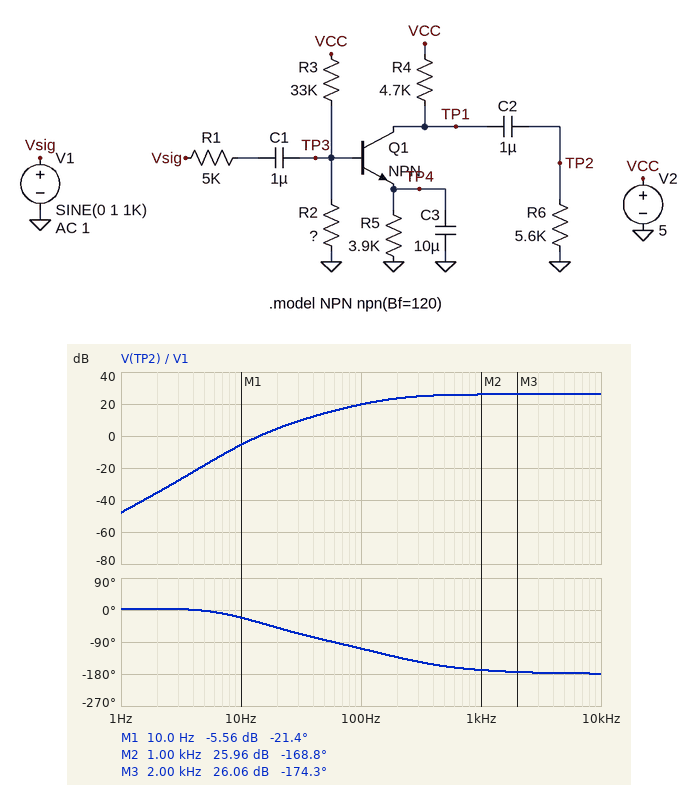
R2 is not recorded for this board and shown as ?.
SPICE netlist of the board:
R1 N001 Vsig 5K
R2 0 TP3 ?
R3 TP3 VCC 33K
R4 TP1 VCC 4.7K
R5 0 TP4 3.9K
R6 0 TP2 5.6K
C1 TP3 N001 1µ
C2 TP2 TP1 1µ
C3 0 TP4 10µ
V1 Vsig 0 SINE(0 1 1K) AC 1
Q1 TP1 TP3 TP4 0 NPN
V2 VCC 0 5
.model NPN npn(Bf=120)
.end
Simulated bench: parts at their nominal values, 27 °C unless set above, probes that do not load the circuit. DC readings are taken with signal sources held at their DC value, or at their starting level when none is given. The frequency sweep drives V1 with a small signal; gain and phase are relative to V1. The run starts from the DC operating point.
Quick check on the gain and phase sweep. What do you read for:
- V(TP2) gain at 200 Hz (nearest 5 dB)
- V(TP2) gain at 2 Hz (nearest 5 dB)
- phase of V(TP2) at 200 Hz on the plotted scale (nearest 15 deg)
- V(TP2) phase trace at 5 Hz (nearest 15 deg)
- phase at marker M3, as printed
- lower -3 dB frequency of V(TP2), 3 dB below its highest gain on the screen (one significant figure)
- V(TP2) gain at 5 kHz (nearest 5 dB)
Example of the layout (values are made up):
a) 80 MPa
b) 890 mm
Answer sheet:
a) 25 dB
b) -35 dB
c) -135 deg
d) 0 deg
e) -174.3 deg
f) 200 Hz
g) 25 dB
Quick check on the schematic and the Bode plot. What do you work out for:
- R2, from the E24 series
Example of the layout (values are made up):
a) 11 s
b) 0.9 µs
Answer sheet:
a) 30 kΩ
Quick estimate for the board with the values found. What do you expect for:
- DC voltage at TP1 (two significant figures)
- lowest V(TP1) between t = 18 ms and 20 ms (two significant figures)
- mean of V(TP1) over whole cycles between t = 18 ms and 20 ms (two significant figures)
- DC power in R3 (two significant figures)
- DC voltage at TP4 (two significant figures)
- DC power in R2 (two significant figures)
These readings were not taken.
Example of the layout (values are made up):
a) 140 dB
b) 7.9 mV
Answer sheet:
a) 3.1 V
b) 1.7 V
c) 3.2 V
d) 220 µW
e) 1.6 V
f) 180 µW
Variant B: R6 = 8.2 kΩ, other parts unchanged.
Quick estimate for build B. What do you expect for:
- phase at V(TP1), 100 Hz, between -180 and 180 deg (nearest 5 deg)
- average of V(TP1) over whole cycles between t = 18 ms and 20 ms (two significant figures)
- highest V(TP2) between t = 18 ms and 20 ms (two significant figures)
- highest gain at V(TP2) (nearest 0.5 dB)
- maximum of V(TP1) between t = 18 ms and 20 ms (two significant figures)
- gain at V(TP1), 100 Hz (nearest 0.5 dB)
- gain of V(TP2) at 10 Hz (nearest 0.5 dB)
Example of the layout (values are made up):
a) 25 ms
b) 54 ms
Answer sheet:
a) -120 deg
b) 3.3 V
c) 1.1 V
d) 27.5 dB
e) 4.4 V
f) 21.5 dB
g) -3.0 dB
